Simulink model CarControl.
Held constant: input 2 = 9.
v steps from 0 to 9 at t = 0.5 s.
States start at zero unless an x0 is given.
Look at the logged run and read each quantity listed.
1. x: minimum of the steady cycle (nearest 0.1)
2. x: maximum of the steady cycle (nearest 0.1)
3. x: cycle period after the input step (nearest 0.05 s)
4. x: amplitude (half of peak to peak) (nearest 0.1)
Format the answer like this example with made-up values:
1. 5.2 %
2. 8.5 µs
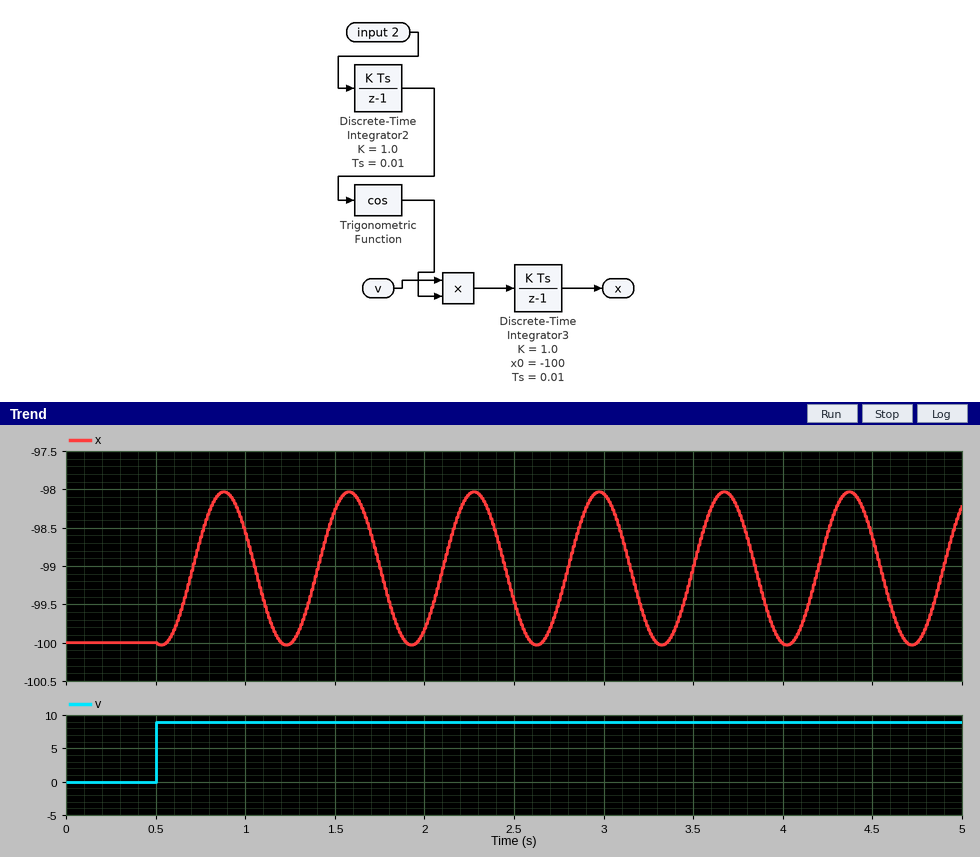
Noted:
1. -100.0
2. -98.0
3. 0.70 s
4. 1.0
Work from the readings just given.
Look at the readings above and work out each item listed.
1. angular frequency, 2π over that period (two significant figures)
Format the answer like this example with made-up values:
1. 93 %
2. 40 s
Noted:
1. 9.0 rad/s
